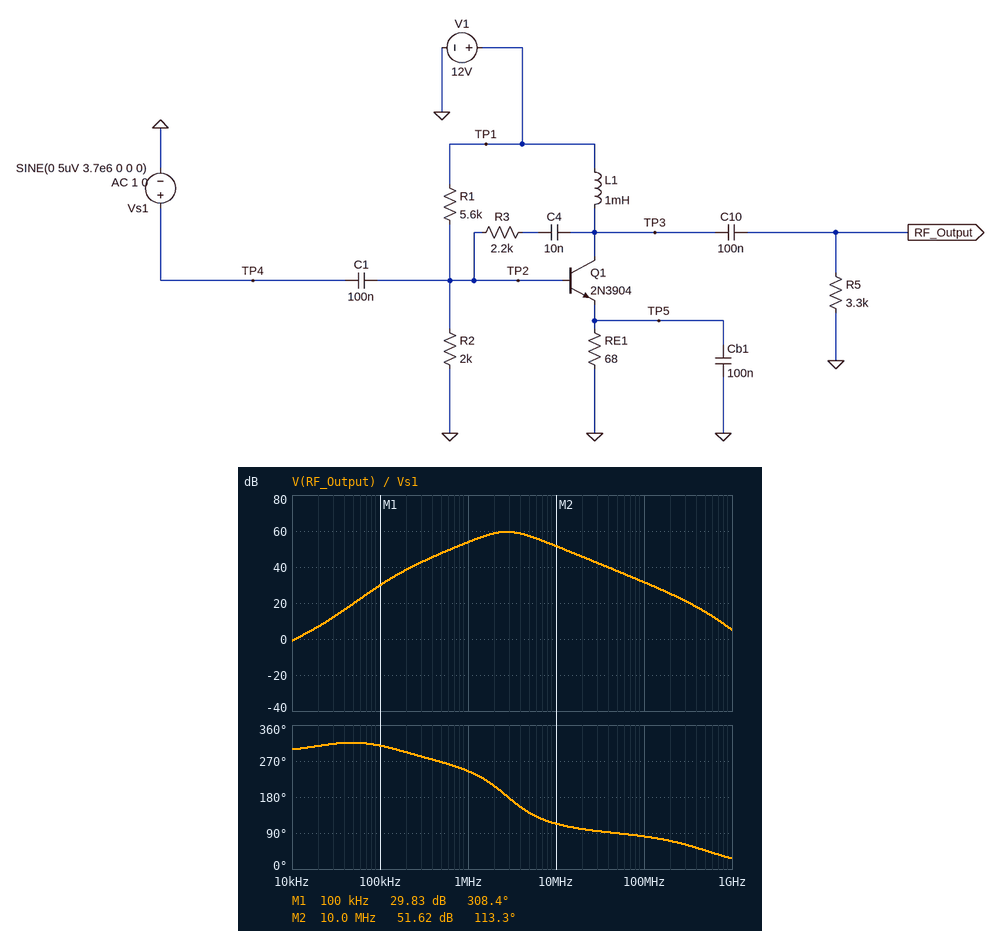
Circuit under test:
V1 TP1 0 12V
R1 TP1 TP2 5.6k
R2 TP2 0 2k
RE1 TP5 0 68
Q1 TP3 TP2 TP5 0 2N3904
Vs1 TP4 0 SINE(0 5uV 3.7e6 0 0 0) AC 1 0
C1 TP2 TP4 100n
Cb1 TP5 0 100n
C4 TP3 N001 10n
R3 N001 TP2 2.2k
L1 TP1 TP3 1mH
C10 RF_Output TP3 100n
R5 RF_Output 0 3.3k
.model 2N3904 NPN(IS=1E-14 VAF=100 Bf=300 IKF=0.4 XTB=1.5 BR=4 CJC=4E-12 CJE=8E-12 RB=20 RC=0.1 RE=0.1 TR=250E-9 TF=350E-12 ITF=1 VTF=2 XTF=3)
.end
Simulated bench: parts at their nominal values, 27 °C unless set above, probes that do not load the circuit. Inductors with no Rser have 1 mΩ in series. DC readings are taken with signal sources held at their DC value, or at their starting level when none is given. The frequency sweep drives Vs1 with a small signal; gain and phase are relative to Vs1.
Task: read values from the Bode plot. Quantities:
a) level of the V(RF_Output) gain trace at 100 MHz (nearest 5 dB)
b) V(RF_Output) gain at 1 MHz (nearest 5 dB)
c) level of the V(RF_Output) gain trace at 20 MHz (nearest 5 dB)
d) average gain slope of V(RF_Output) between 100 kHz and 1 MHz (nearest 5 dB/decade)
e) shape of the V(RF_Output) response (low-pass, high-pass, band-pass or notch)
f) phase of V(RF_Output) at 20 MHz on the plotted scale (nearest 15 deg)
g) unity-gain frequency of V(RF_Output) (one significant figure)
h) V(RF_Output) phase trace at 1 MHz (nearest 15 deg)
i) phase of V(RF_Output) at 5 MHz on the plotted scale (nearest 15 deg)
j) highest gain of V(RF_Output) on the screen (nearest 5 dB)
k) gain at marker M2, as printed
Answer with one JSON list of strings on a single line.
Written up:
["30 dB", "55 dB", "45 dB", "25 dB/decade", "band-pass", "105 deg", "10 kHz", "240 deg", "135 deg", "60 dB", "51.62 dB"]
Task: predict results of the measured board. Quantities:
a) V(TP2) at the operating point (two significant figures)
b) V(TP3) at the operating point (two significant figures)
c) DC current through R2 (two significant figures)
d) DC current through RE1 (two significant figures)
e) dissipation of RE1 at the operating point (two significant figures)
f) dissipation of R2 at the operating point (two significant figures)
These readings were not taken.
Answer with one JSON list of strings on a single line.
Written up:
["3.0 V", "12 V", "1.5 mA", "33 mA", "74 mW", "4.5 mW"]
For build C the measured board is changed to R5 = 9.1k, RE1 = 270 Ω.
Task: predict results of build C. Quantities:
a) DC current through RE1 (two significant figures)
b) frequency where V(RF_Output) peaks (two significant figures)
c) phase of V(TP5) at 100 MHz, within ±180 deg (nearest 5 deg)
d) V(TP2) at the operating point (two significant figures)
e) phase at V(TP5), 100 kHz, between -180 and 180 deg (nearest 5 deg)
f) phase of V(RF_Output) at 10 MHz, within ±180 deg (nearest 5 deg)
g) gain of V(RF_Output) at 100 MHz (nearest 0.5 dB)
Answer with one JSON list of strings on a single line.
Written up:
["8.9 mA", "2.6 MHz", "-110 deg", "3.1 V", "-20 deg", "130 deg", "31.0 dB"]
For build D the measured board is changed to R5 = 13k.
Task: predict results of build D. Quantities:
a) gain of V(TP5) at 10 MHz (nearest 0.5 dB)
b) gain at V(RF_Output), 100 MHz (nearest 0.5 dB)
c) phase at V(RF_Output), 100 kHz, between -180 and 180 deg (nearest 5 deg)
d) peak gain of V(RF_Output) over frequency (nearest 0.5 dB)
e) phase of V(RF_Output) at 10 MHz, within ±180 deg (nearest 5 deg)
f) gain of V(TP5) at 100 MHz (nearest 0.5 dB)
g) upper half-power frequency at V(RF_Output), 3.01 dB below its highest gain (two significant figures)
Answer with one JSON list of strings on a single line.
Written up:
["-29.0 dB", "32.0 dB", "-45 deg", "61.5 dB", "110 deg", "-62.0 dB", "4.7 MHz"]
